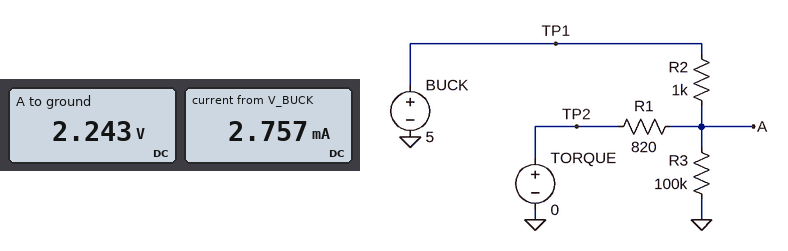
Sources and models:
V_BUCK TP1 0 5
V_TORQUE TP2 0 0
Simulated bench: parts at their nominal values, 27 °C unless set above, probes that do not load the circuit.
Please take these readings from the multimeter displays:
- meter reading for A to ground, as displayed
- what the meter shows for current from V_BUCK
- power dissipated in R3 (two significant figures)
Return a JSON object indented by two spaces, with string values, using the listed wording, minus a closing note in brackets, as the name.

{
  "meter reading for A to ground, as displayed": "2.243 V",
  "what the meter shows for current from V_BUCK": "2.757 mA",
  "power dissipated in R3": "50 µW"
}
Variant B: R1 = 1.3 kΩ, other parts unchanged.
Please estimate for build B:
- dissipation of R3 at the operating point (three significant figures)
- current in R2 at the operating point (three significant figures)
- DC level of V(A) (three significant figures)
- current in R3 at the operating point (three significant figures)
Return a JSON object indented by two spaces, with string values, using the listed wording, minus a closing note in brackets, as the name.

{
  "dissipation of R3 at the operating point": "79.0 µW",
  "current in R2 at the operating point": "2.19 mA",
  "DC level of V(A)": "2.81 V",
  "current in R3 at the operating point": "28.1 µA"
}
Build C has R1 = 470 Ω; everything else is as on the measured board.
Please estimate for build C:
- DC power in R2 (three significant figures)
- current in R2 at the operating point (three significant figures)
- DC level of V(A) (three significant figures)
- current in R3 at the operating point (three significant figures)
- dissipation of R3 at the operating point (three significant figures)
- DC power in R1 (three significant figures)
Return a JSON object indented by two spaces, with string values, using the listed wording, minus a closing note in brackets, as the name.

{
  "DC power in R2": "11.6 mW",
  "current in R2 at the operating point": "3.41 mA",
  "DC level of V(A)": "1.59 V",
  "current in R3 at the operating point": "15.9 µA",
  "dissipation of R3 at the operating point": "25.4 µW",
  "DC power in R1": "5.40 mW"
}
